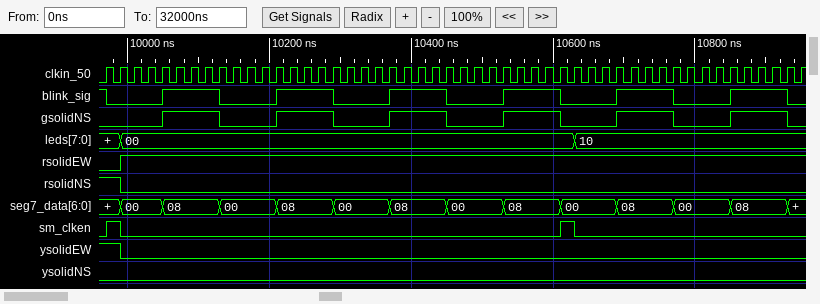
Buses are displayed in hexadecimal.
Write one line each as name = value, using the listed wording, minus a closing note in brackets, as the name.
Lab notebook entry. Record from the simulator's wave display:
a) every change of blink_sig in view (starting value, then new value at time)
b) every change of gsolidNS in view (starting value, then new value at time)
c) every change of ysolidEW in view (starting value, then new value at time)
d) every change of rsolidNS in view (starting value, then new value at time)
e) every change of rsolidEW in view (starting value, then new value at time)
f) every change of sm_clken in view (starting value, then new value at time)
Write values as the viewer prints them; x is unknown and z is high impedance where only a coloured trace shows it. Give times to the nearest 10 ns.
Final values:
every change of blink_sig in view = 1, 0 at 9970 ns, 1 at 10050 ns, 0 at 10130 ns, 1 at 10210 ns, 0 at 10290 ns, 1 at 10370 ns, 0 at 10450 ns, 1 at 10530 ns, 0 at 10610 ns, 1 at 10690 ns, 0 at 10770 ns, 1 at 10850 ns, 0 at 10930 ns
every change of gsolidNS in view = 0, 1 at 10050 ns, 0 at 10130 ns, 1 at 10210 ns, 0 at 10290 ns, 1 at 10370 ns, 0 at 10450 ns, 1 at 10530 ns, 0 at 10610 ns, 1 at 10690 ns, 0 at 10770 ns, 1 at 10850 ns, 0 at 10930 ns
every change of ysolidEW in view = 1, 0 at 9990 ns
every change of rsolidNS in view = 1, 0 at 9990 ns
every change of rsolidEW in view = 0, 1 at 9990 ns
every change of sm_clken in view = 0, 1 at 9970 ns, 0 at 9990 ns, 1 at 10610 ns, 0 at 10630 ns
